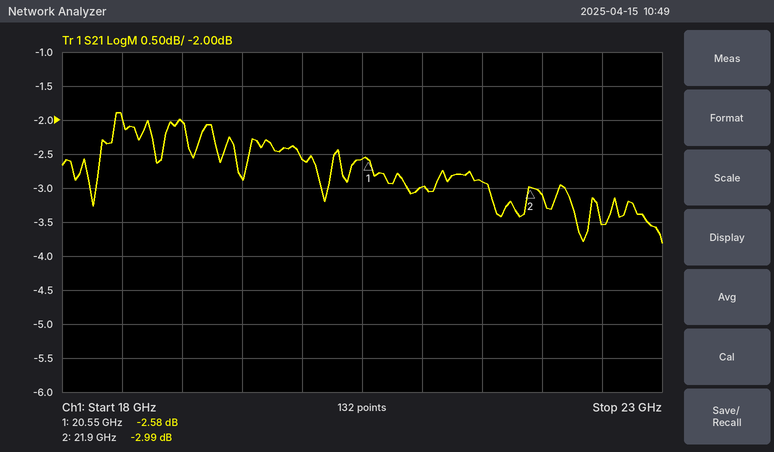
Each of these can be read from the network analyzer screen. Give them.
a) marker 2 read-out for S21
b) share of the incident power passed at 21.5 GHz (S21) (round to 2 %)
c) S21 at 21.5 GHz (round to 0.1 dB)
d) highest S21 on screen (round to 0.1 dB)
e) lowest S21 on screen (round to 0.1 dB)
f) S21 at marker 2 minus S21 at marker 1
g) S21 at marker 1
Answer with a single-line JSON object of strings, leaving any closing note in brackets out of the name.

{"marker 2 read-out for S21": "-2.99 dB", "share of the incident power passed at 21.5 GHz (S21)": "52 %", "S21 at 21.5 GHz": "-2.9 dB", "highest S21 on screen": "-1.9 dB", "lowest S21 on screen": "-3.8 dB", "S21 at marker 2 minus S21 at marker 1": "-0.41 dB", "S21 at marker 1": "-2.58 dB"}
